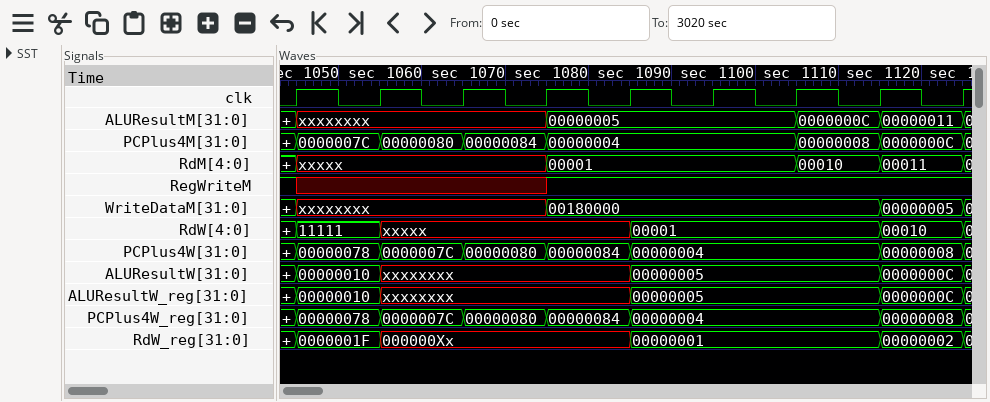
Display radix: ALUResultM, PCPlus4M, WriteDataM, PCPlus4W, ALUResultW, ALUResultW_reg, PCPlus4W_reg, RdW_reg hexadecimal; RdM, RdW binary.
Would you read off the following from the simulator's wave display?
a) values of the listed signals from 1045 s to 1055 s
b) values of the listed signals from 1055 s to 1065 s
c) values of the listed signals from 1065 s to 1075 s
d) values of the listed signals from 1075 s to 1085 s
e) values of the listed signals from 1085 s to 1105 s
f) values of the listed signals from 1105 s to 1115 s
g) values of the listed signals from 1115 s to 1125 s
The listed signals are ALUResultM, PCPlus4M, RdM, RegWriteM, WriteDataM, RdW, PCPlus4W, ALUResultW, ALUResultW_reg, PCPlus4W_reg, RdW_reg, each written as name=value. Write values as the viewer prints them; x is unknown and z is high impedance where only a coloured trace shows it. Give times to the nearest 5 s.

ALUResultM=xxxxxxxx, PCPlus4M=0000007C, RdM=xxxxx, RegWriteM=x, WriteDataM=xxxxxxxx, RdW=11111, PCPlus4W=00000078, ALUResultW=00000010, ALUResultW_reg=00000010, PCPlus4W_reg=00000078, RdW_reg=0000001F
ALUResultM=xxxxxxxx, PCPlus4M=00000080, RdM=xxxxx, RegWriteM=x, WriteDataM=xxxxxxxx, RdW=xxxxx, PCPlus4W=0000007C, ALUResultW=xxxxxxxx, ALUResultW_reg=xxxxxxxx, PCPlus4W_reg=0000007C, RdW_reg=000000Xx
ALUResultM=xxxxxxxx, PCPlus4M=00000084, RdM=xxxxx, RegWriteM=x, WriteDataM=xxxxxxxx, RdW=xxxxx, PCPlus4W=00000080, ALUResultW=xxxxxxxx, ALUResultW_reg=xxxxxxxx, PCPlus4W_reg=00000080, RdW_reg=000000Xx
ALUResultM=00000005, PCPlus4M=00000004, RdM=00001, RegWriteM=1, WriteDataM=00180000, RdW=xxxxx, PCPlus4W=00000084, ALUResultW=xxxxxxxx, ALUResultW_reg=xxxxxxxx, PCPlus4W_reg=00000084, RdW_reg=000000Xx
ALUResultM=00000005, PCPlus4M=00000004, RdM=00001, RegWriteM=1, WriteDataM=00180000, RdW=00001, PCPlus4W=00000004, ALUResultW=00000005, ALUResultW_reg=00000005, PCPlus4W_reg=00000004, RdW_reg=00000001
ALUResultM=0000000C, PCPlus4M=00000008, RdM=00010, RegWriteM=1, WriteDataM=00180000, RdW=00001, PCPlus4W=00000004, ALUResultW=00000005, ALUResultW_reg=00000005, PCPlus4W_reg=00000004, RdW_reg=00000001
ALUResultM=00000011, PCPlus4M=0000000C, RdM=00011, RegWriteM=1, WriteDataM=00000005, RdW=00010, PCPlus4W=00000008, ALUResultW=0000000C, ALUResultW_reg=0000000C, PCPlus4W_reg=00000008, RdW_reg=00000002
